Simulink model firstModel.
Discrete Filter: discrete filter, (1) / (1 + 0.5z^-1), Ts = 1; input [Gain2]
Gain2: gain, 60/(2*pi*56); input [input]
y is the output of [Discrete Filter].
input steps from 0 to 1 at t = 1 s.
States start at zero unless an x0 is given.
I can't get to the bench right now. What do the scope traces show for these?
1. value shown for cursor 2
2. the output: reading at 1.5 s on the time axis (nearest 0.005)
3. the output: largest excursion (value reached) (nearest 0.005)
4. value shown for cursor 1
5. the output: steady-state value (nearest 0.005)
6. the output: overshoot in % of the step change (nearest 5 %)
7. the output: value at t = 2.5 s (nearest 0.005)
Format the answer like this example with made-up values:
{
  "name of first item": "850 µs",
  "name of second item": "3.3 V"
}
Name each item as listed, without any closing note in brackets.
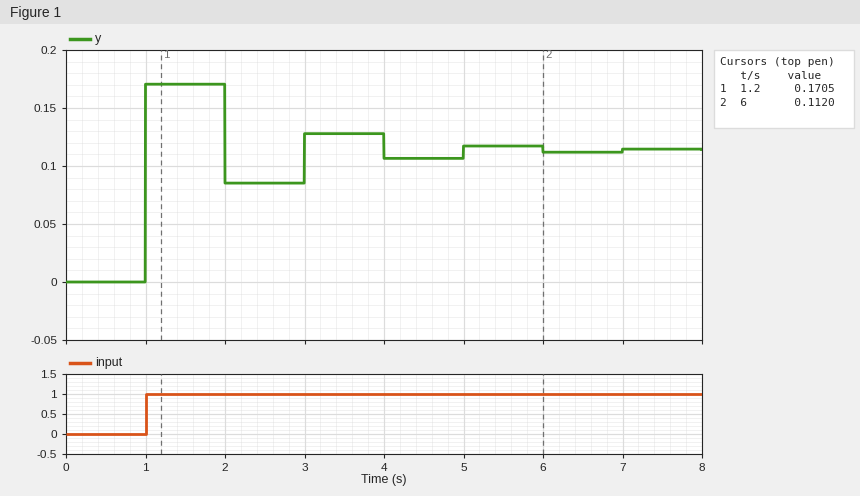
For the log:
{
  "value shown for cursor 2": "0.1120",
  "the output: reading at 1.5 s on the time axis": "0.170",
  "the output: largest excursion (value reached)": "0.170",
  "value shown for cursor 1": "0.1705",
  "the output: steady-state value": "0.115",
  "the output: overshoot in % of the step change": "50 %",
  "the output: value at t = 2.5 s": "0.085"
}
